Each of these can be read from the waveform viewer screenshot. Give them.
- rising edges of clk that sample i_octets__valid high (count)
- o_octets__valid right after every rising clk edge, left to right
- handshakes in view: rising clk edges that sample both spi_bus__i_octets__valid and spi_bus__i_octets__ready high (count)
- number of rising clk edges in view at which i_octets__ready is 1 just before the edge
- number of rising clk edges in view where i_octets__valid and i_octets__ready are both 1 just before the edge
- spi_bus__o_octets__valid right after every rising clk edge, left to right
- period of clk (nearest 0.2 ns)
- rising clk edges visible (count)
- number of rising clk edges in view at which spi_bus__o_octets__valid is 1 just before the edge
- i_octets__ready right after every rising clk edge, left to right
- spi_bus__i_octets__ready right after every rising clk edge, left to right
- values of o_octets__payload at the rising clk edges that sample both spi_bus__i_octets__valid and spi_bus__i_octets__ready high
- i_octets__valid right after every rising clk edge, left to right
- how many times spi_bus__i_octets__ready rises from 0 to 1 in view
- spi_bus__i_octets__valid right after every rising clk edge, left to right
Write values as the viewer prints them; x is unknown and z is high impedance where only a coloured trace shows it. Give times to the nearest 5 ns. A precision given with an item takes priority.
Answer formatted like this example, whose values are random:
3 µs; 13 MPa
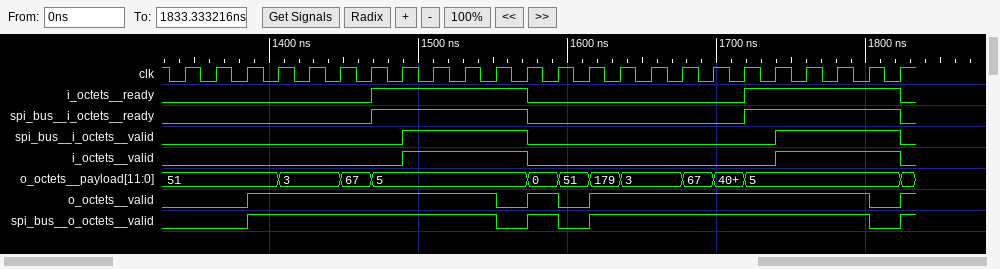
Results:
8; 0 0 1 1 1 1 1 1 1 1 0 1 0 1 1 1 1 1 1 1 1 1 0 1; 8; 10; 8; 0 0 1 1 1 1 1 1 1 1 0 1 0 1 1 1 1 1 1 1 1 1 0 1; 20.8 ns; 24; 18; 0 0 0 0 0 0 1 1 1 1 1 0 0 0 0 0 0 0 1 1 1 1 1 0; 0 0 0 0 0 0 1 1 1 1 1 0 0 0 0 0 0 0 1 1 1 1 1 0; 5, 5, 5, 5, 5, 5, 5, 5; 0 0 0 0 0 0 0 1 1 1 1 0 0 0 0 0 0 0 0 1 1 1 1 0; 2; 0 0 0 0 0 0 0 1 1 1 1 0 0 0 0 0 0 0 0 1 1 1 1 0
